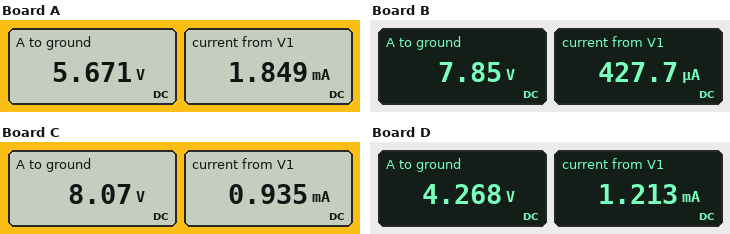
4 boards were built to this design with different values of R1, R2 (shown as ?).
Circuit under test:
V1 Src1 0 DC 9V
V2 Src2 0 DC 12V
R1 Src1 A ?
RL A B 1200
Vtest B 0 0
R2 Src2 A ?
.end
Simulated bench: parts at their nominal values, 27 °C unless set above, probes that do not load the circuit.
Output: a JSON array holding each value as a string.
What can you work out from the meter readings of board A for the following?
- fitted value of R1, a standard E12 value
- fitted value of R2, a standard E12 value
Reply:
["1.8 kΩ", "2.2 kΩ"]
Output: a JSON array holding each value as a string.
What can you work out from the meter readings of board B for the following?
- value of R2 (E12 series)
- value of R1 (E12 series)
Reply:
["680 Ω", "2.7 kΩ"]
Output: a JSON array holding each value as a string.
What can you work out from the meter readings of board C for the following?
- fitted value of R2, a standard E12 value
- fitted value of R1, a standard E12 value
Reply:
["680 Ω", "1 kΩ"]
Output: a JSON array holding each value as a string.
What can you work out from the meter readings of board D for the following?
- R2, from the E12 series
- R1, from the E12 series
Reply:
["3.3 kΩ", "3.9 kΩ"]
